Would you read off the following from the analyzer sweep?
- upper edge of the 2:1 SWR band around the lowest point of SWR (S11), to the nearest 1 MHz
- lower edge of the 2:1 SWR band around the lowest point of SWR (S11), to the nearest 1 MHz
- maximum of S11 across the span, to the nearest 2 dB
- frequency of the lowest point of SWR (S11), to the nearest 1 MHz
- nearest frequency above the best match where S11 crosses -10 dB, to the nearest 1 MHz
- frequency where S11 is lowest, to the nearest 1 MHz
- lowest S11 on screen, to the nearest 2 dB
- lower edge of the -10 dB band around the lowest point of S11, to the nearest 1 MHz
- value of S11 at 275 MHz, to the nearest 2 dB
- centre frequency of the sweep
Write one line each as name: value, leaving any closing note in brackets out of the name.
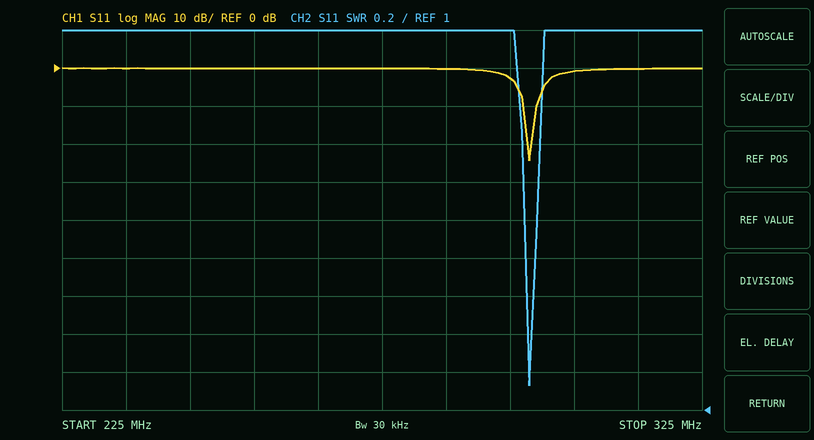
upper edge of the 2:1 SWR band around the lowest point of SWR (S11), to the nearest 1 MHz: 299 MHz
lower edge of the 2:1 SWR band around the lowest point of SWR (S11), to the nearest 1 MHz: 297 MHz
maximum of S11 across the span, to the nearest 2 dB: 0 dB
frequency of the lowest point of SWR (S11), to the nearest 1 MHz: 298 MHz
nearest frequency above the best match where S11 crosses -10 dB, to the nearest 1 MHz: 299 MHz
frequency where S11 is lowest, to the nearest 1 MHz: 298 MHz
lowest S11 on screen, to the nearest 2 dB: -24 dB
lower edge of the -10 dB band around the lowest point of S11, to the nearest 1 MHz: 297 MHz
value of S11 at 275 MHz, to the nearest 2 dB: 0 dB
centre frequency of the sweep: 275 MHz
